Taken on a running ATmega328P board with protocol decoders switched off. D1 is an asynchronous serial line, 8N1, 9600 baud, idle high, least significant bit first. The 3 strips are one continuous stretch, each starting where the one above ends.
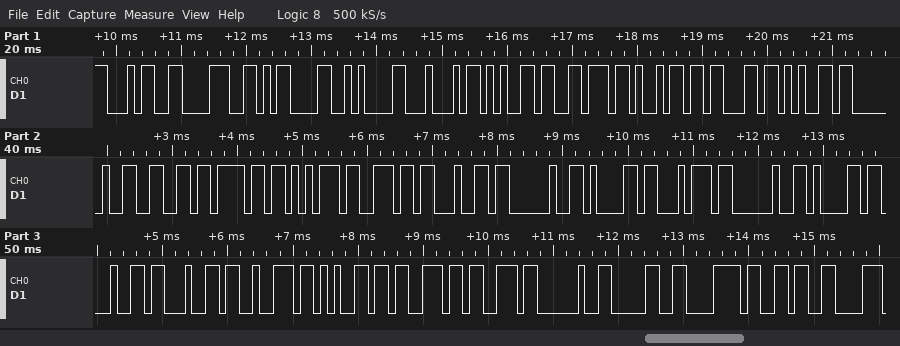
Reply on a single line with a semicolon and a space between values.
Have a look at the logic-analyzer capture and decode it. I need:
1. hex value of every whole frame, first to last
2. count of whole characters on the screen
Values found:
0x34 0x38 0x0D 0x0A 0x44 0x65 0x76 0x69 0x63 0x65 0x20 0x66 0x6F 0x75 0x6E 0x64 0x20 0x61 0x74 0x20 0x61 0x64 0x64 0x72 0x65 0x73 0x73 0x20 0x30 0x78 0x36; 31
